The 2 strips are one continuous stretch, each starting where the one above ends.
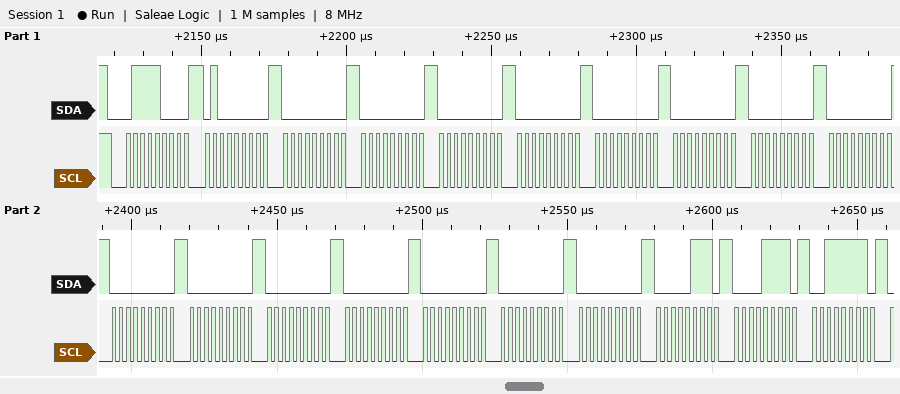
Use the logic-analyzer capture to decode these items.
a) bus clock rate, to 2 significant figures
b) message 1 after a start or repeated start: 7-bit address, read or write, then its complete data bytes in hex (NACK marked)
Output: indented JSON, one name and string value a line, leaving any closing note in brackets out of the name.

{
  "bus clock rate, to 2 significant figures": "400 kHz",
  "message 1 after a start or repeated start: 7-bit address, read or write, then its complete data bytes in hex": "0x3C write: 40 00 00 00 00 00 00 00 00 00 00 00 00 00 00 00 07 0F 3F"
}
